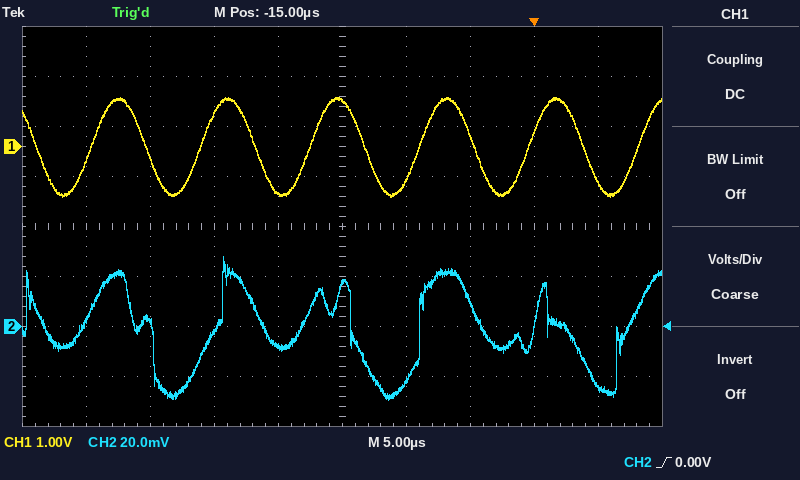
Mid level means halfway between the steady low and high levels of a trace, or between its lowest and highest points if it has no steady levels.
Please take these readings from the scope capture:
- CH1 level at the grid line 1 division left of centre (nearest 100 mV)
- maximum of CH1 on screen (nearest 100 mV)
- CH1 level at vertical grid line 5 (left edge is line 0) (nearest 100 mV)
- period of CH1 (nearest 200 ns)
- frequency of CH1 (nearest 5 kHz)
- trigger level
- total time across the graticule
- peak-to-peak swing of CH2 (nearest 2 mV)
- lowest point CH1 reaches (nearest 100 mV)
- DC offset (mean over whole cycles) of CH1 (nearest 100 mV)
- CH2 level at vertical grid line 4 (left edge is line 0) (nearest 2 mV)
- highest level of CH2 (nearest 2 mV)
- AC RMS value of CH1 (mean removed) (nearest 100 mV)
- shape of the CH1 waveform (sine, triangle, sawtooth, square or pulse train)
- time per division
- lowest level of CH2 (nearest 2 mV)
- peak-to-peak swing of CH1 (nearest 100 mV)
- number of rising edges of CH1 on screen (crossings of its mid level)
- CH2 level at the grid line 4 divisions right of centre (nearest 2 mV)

-900 mV
1.0 V
900 mV
8.6 µs
115 kHz
0.00 V
50 µs
58 mV
-1.0 V
0.0 V
-8 mV
28 mV
700 mV
sine
5 µs
-30 mV
2.0 V
6
-24 mV
